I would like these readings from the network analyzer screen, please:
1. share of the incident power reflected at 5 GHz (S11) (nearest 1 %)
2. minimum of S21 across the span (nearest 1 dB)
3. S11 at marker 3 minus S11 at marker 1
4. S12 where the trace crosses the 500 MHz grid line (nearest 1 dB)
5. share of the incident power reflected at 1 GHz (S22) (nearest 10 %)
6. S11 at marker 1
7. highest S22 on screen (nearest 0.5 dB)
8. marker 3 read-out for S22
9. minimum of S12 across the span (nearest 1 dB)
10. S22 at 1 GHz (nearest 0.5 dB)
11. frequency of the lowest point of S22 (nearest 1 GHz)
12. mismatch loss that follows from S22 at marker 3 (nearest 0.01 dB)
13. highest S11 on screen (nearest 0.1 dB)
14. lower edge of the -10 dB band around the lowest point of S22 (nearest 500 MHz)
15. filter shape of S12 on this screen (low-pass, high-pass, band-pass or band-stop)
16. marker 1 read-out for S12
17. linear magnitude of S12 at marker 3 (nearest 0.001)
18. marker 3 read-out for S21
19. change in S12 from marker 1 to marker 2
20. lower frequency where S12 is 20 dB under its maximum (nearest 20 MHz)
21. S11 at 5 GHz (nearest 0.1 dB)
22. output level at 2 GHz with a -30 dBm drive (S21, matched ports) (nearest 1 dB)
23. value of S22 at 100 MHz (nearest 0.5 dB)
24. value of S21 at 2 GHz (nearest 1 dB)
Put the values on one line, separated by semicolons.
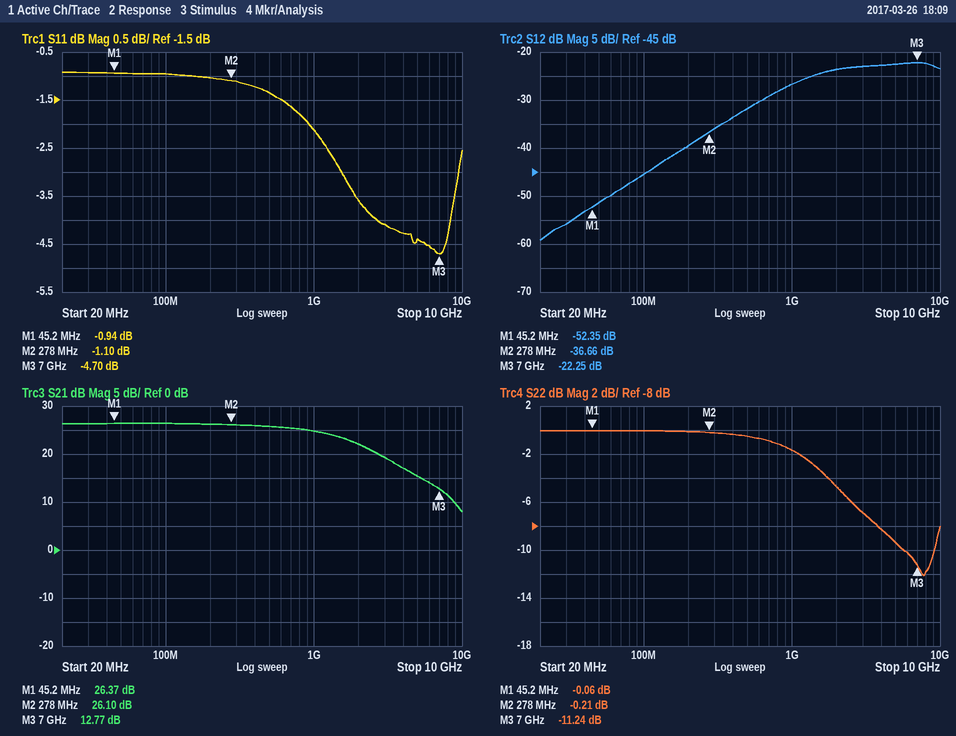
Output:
36 %; 8 dB; -3.76 dB; -32 dB; 70 %; -0.94 dB; 0.0 dB; -11.24 dB; -59 dB; -1.5 dB; 8 GHz; 0.34 dB; -0.9 dB; 5.5 GHz; high-pass; -52.35 dB; 0.077; 12.77 dB; 15.69 dB; 140 MHz; -4.4 dB; -8 dBm; 0.0 dB; 22 dB
